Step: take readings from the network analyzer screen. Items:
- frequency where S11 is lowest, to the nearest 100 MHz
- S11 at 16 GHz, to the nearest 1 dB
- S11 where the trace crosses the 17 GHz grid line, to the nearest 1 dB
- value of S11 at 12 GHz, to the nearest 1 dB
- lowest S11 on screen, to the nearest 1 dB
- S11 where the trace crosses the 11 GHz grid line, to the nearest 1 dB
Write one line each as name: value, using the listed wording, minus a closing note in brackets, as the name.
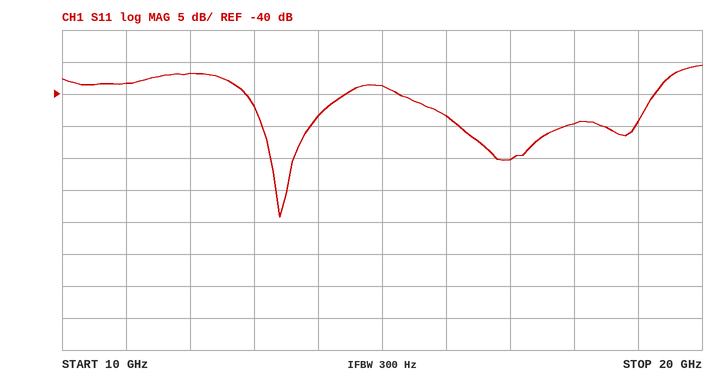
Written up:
frequency where S11 is lowest, to the nearest 100 MHz: 13.4 GHz
S11 at 16 GHz, to the nearest 1 dB: -43 dB
S11 where the trace crosses the 17 GHz grid line, to the nearest 1 dB: -50 dB
value of S11 at 12 GHz, to the nearest 1 dB: -37 dB
lowest S11 on screen, to the nearest 1 dB: -59 dB
S11 where the trace crosses the 11 GHz grid line, to the nearest 1 dB: -38 dB
